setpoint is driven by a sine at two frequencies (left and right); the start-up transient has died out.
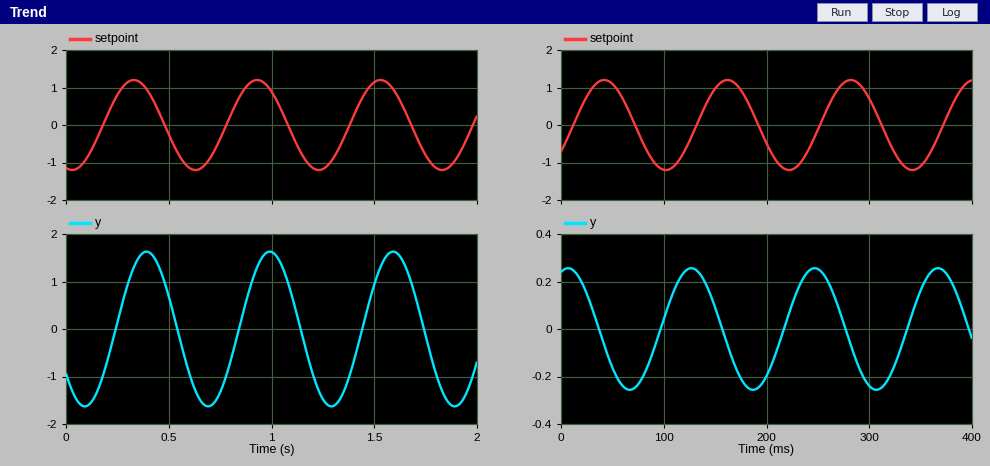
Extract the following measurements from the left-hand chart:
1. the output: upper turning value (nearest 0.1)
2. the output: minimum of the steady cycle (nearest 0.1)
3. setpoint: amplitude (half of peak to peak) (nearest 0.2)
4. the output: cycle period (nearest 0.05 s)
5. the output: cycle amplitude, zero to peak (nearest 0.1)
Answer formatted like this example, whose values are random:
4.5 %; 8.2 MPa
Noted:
1.6; -1.6; 1.2; 0.60 s; 1.6
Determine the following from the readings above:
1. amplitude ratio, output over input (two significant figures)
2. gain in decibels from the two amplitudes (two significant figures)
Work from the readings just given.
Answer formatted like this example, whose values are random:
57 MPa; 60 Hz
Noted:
1.3; 2.5 dB
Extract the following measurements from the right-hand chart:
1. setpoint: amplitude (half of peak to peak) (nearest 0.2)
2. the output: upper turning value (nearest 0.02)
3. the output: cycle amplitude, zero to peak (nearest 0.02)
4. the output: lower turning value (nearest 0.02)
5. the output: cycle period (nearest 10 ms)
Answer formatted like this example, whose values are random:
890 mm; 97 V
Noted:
1.2; 0.26; 0.26; -0.26; 120 ms
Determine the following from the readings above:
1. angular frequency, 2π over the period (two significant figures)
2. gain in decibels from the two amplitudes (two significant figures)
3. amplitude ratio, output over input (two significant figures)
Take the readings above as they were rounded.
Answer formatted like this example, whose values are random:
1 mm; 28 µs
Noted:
0.052 rad/ms; -13 dB; 0.22
